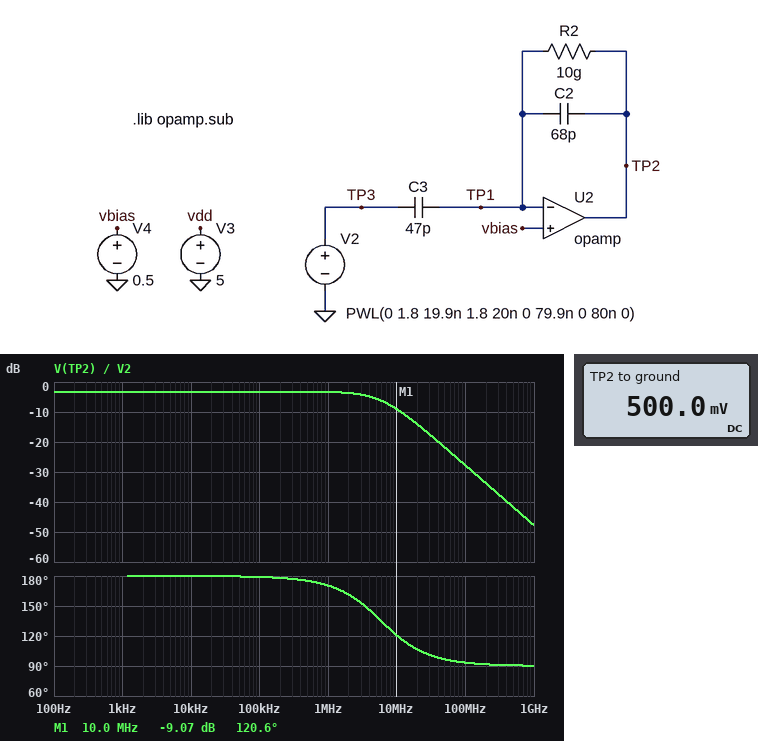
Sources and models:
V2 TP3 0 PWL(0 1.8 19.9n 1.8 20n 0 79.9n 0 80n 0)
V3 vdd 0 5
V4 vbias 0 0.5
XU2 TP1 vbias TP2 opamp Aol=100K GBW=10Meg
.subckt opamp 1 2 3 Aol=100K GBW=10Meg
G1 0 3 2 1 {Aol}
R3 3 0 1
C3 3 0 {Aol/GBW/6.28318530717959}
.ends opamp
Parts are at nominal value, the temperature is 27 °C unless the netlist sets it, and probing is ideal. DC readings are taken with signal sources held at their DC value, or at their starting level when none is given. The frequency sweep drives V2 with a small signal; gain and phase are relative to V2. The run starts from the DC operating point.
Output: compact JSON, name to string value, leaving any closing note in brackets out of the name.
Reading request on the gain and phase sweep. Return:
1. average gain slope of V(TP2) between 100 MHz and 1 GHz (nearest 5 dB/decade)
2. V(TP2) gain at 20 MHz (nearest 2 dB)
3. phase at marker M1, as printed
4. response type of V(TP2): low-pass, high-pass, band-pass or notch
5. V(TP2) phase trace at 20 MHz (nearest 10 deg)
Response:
{"average gain slope of V(TP2) between 100 MHz and 1 GHz": "-20 dB/decade", "V(TP2) gain at 20 MHz": "-14 dB", "phase at marker M1, as printed": "120.6 deg", "response type of V(TP2): low-pass, high-pass, band-pass or notch": "low-pass", "V(TP2) phase trace at 20 MHz": "110 deg"}
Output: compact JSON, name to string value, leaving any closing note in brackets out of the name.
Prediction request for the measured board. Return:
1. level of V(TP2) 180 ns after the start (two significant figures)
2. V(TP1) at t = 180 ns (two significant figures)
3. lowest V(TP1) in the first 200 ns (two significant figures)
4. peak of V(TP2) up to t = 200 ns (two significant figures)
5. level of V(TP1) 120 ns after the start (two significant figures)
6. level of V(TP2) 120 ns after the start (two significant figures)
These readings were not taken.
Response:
{"level of V(TP2) 180 ns after the start": "1.7 V", "V(TP1) at t = 180 ns": "500 mV", "lowest V(TP1) in the first 200 ns": "-230 mV", "peak of V(TP2) up to t = 200 ns": "1.7 V", "level of V(TP1) 120 ns after the start": "480 mV", "level of V(TP2) 120 ns after the start": "1.7 V"}
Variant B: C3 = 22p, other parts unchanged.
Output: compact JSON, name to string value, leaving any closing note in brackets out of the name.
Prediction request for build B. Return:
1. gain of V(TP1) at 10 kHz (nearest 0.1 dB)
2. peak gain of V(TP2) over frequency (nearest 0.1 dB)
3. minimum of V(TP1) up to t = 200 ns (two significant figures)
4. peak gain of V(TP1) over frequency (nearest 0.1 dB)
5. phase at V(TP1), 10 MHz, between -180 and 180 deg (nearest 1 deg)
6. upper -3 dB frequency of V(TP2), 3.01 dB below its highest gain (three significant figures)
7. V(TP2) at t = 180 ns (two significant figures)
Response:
{"gain of V(TP1) at 10 kHz": "-69.8 dB", "peak gain of V(TP2) over frequency": "-9.8 dB", "minimum of V(TP1) up to t = 200 ns": "61 mV", "peak gain of V(TP1) over frequency": "-12.2 dB", "phase at V(TP1), 10 MHz, between -180 and 180 deg": "37 deg", "upper -3 dB frequency of V(TP2), 3.01 dB below its highest gain": "7.56 MHz", "V(TP2) at t = 180 ns": "1.1 V"}
